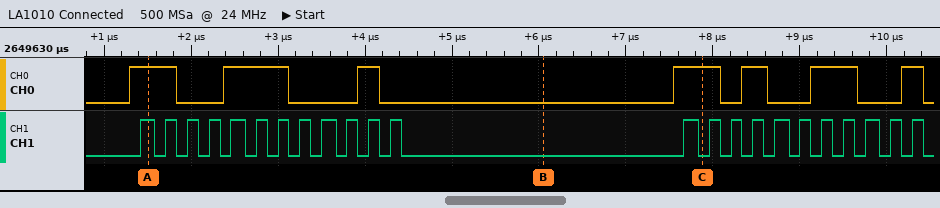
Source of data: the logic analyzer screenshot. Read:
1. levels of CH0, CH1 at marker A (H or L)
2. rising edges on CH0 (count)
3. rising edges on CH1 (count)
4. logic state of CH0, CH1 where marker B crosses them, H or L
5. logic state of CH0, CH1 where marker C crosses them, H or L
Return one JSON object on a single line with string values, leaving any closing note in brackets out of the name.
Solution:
{"levels of CH0, CH1 at marker A": "CH0=H, CH1=H", "rising edges on CH0": "7", "rising edges on CH1": "23", "logic state of CH0, CH1 where marker B crosses them, H or L": "CH0=L, CH1=L", "logic state of CH0, CH1 where marker C crosses them, H or L": "CH0=H, CH1=L"}
